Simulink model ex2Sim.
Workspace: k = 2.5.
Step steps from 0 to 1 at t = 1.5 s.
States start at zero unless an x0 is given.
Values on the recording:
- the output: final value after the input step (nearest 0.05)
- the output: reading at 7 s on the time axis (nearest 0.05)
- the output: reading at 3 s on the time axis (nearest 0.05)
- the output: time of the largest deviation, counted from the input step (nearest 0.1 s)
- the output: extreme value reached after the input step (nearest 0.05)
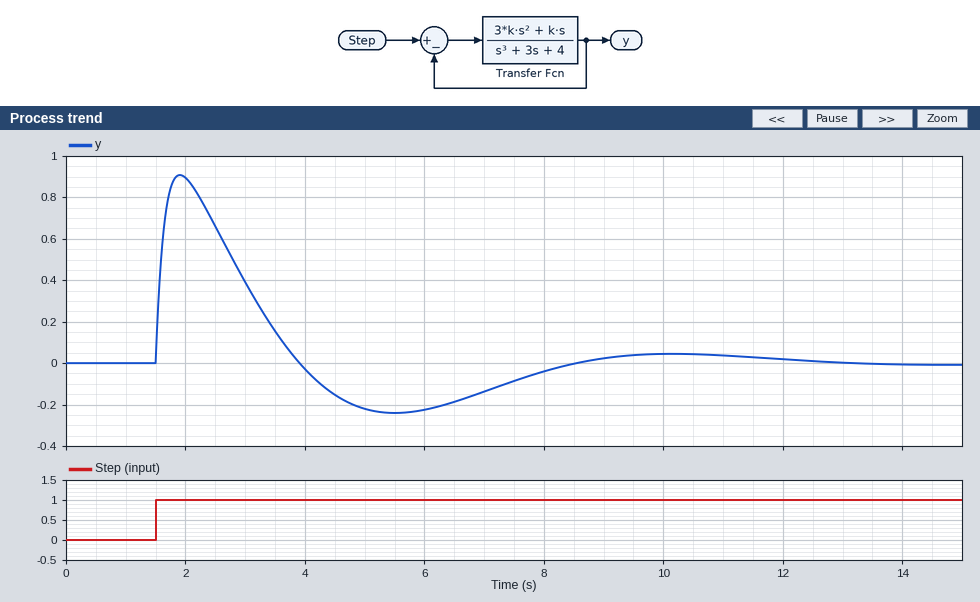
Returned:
0.00
-0.15
0.40
0.4 s
0.90
